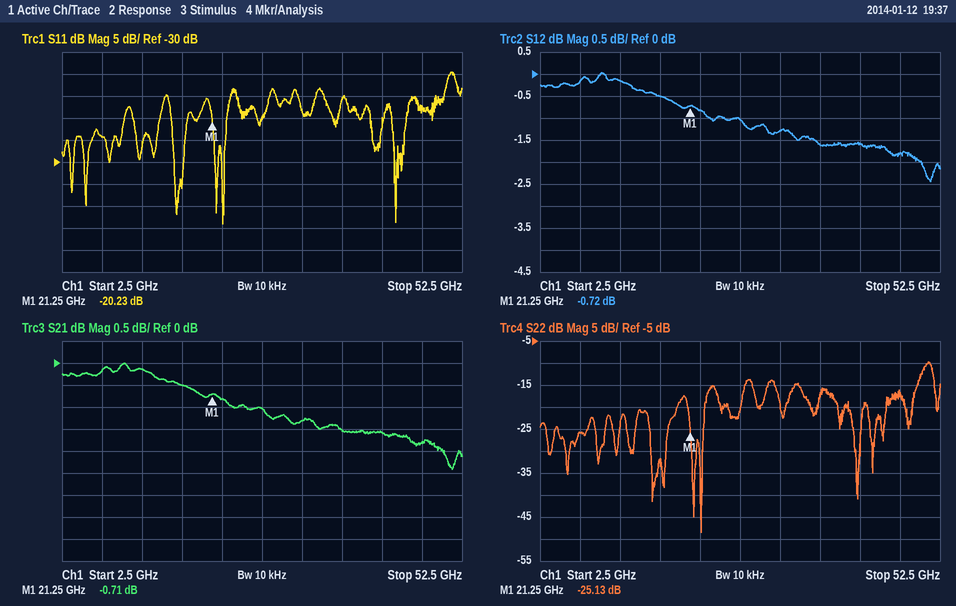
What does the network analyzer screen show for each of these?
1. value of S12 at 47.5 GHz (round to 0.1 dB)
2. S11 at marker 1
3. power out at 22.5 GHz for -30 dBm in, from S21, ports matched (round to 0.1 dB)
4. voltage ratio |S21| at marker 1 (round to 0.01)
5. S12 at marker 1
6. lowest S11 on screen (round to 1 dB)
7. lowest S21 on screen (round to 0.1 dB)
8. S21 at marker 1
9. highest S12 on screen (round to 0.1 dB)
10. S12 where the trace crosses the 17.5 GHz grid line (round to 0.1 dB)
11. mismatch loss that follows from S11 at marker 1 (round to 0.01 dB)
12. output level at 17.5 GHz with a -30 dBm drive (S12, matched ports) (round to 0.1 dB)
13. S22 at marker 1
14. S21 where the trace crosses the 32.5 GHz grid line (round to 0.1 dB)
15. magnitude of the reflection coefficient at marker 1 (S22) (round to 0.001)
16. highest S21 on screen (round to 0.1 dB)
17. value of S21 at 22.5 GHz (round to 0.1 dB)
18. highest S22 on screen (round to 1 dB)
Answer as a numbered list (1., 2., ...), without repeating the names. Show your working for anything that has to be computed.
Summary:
1. -1.8 dB
2. -20.23 dB
3. -30 dBm + (-0.8 dB) = -30.8 dBm
4. 10^(-0.71/20) ≈ 0.92
5. -0.72 dB
6. -44 dB
7. -2.4 dB
8. -0.71 dB
9. 0.0 dB
10. -0.5 dB
11. −10 log10(1 − 10^(-20.23/10)) ≈ 0.04 dB
12. -30 dBm + (-0.5 dB) = -30.5 dBm
13. -25.13 dB
14. -1.3 dB
15. 10^(-25.13/20) ≈ 0.055
16. 0.0 dB
17. -0.8 dB
18. -10 dB
